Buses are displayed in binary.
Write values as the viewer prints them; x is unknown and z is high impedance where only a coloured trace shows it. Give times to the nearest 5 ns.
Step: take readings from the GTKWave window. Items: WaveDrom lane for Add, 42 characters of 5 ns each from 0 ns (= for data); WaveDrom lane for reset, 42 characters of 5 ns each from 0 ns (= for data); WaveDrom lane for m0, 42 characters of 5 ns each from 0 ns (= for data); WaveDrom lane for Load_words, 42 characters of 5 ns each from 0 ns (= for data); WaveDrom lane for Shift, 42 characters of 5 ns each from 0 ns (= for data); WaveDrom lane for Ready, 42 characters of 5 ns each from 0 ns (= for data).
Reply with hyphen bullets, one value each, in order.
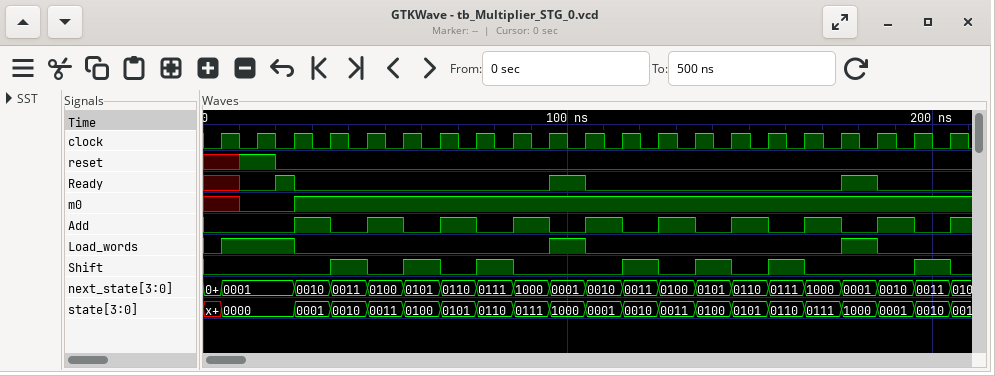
- {name: 'Add', wave: '0....1.0.1.0.1.0.1.0.1.0.1.0.1.0.1.0.1.0.1'}
- {name: 'reset', wave: 'x.1.0.....................................'}
- {name: 'm0', wave: 'x.0..1....................................'}
- {name: 'Load_words', wave: '01...0.............1.0.............1.0....'}
- {name: 'Shift', wave: '0......1.0.1.0.1.0.....1.0.1.0.1.0.....1.0'}
- {name: 'Ready', wave: 'x.0.10.............1.0.............1.0....'}
